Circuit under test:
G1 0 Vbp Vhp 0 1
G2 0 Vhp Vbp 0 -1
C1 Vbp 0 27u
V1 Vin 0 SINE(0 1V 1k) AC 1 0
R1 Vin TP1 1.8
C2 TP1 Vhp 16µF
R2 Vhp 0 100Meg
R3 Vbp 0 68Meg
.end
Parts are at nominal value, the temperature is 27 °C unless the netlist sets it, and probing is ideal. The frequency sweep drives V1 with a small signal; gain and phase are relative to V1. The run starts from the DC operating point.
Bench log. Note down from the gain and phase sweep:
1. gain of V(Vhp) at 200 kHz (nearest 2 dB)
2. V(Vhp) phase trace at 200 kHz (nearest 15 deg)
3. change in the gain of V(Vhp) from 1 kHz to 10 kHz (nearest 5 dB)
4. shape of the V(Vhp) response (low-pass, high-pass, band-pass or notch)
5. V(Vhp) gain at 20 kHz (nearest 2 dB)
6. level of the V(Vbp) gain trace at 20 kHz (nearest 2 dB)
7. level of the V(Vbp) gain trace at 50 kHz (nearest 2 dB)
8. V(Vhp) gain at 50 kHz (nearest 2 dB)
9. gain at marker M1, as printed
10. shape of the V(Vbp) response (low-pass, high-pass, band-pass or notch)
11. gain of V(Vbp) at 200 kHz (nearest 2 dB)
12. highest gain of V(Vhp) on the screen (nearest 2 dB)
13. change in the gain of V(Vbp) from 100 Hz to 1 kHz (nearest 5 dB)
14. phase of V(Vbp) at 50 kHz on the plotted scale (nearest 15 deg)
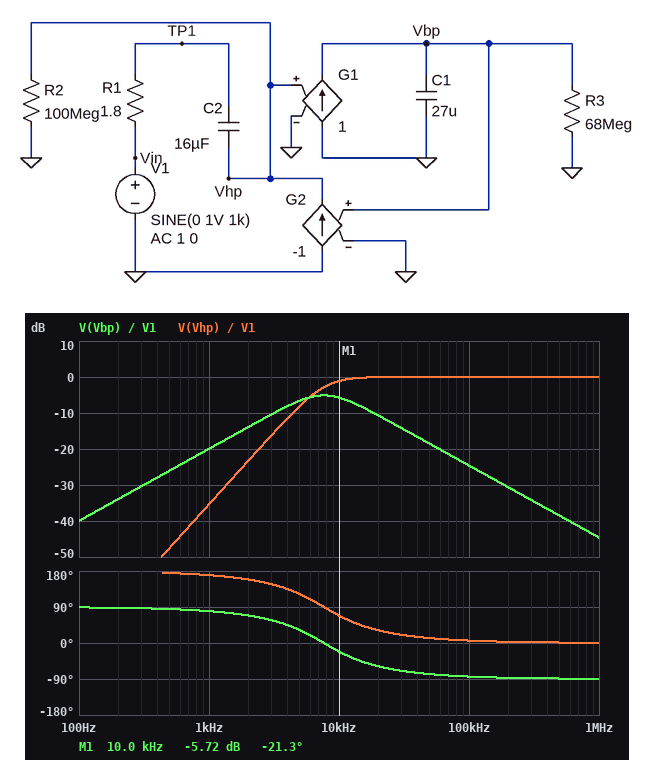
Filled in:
0 dB
0 deg
35 dB
high-pass
0 dB
-10 dB
-18 dB
0 dB
-5.72 dB
band-pass
-30 dB
0 dB
20 dB
-75 deg
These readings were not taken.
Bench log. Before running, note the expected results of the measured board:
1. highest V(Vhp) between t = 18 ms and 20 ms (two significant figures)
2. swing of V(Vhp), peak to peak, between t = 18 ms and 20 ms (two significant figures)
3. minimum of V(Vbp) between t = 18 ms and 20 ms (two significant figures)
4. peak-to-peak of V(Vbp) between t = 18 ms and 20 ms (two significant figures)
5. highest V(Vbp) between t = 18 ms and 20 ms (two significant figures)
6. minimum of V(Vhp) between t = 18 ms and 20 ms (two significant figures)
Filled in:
17 mV
34 mV
-100 mV
200 mV
100 mV
-17 mV
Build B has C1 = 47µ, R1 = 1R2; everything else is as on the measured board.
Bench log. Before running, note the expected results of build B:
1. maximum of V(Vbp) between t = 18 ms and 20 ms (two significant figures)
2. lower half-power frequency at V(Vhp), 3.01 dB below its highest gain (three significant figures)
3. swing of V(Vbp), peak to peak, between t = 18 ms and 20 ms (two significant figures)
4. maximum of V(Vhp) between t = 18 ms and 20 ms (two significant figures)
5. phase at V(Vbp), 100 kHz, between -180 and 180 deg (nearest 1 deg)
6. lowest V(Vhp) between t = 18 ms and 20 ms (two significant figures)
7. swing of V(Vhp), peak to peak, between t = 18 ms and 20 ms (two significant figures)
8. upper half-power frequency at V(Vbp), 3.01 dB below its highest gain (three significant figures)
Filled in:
100 mV
4.89 kHz
210 mV
30 mV
-88 deg
-30 mV
61 mV
8.18 kHz
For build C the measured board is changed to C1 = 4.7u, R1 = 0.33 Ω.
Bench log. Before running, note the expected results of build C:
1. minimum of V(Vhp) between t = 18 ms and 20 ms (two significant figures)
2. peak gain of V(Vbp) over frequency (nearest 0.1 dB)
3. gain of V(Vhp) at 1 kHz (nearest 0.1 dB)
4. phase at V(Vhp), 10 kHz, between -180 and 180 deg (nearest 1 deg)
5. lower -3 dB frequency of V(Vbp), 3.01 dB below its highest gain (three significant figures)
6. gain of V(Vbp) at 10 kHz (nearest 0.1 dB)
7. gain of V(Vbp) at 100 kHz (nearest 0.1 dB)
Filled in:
-3.0 mV
9.6 dB
-50.5 dB
155 deg
13.6 kHz
2.2 dB
-9.2 dB
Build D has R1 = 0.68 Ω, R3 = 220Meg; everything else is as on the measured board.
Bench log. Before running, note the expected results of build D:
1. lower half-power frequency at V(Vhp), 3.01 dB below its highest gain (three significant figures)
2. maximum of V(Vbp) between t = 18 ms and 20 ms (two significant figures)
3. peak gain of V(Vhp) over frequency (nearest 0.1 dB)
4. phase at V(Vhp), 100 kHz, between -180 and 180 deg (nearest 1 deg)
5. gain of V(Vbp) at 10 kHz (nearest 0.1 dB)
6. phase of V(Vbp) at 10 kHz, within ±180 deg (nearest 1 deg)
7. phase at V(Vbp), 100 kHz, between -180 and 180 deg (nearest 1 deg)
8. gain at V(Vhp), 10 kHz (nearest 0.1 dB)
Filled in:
6.55 kHz
100 mV
5.9 dB
2 deg
0.2 dB
-46 deg
-88 deg
4.8 dB
